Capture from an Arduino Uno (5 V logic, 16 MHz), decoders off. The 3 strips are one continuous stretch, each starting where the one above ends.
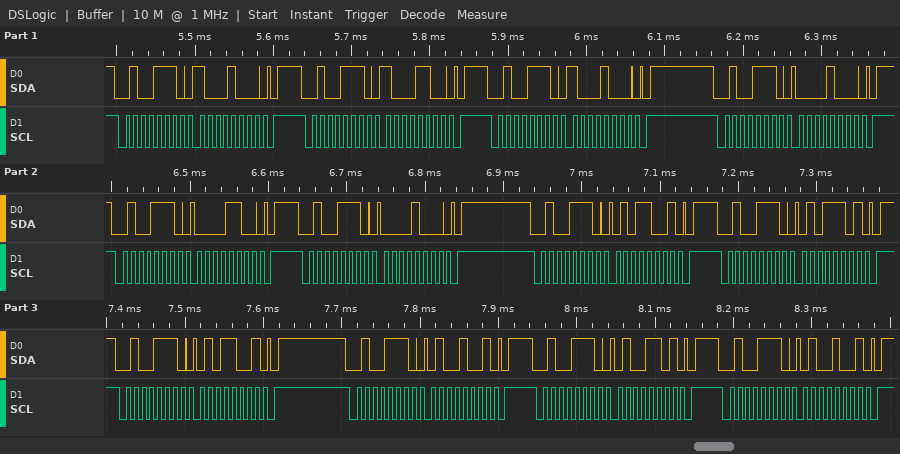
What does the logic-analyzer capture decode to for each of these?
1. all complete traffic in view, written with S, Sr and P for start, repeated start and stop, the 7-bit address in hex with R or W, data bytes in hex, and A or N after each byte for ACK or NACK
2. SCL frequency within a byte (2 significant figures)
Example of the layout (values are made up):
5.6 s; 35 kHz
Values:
S 27W A 88 A P S 27W A 8C A P S 27W A 88 A P S 27W A 08 A P S 27W A 0C A P S 27W A 08 A P S 27W A 59 A P S 27W A 5D A P S 27W A 59 A P S 27W A 49 A P S 27W A 4D A P S 27W A 49 A P; 100 kHz
